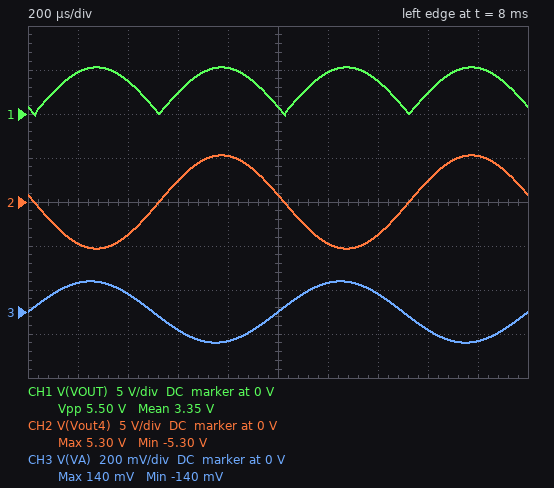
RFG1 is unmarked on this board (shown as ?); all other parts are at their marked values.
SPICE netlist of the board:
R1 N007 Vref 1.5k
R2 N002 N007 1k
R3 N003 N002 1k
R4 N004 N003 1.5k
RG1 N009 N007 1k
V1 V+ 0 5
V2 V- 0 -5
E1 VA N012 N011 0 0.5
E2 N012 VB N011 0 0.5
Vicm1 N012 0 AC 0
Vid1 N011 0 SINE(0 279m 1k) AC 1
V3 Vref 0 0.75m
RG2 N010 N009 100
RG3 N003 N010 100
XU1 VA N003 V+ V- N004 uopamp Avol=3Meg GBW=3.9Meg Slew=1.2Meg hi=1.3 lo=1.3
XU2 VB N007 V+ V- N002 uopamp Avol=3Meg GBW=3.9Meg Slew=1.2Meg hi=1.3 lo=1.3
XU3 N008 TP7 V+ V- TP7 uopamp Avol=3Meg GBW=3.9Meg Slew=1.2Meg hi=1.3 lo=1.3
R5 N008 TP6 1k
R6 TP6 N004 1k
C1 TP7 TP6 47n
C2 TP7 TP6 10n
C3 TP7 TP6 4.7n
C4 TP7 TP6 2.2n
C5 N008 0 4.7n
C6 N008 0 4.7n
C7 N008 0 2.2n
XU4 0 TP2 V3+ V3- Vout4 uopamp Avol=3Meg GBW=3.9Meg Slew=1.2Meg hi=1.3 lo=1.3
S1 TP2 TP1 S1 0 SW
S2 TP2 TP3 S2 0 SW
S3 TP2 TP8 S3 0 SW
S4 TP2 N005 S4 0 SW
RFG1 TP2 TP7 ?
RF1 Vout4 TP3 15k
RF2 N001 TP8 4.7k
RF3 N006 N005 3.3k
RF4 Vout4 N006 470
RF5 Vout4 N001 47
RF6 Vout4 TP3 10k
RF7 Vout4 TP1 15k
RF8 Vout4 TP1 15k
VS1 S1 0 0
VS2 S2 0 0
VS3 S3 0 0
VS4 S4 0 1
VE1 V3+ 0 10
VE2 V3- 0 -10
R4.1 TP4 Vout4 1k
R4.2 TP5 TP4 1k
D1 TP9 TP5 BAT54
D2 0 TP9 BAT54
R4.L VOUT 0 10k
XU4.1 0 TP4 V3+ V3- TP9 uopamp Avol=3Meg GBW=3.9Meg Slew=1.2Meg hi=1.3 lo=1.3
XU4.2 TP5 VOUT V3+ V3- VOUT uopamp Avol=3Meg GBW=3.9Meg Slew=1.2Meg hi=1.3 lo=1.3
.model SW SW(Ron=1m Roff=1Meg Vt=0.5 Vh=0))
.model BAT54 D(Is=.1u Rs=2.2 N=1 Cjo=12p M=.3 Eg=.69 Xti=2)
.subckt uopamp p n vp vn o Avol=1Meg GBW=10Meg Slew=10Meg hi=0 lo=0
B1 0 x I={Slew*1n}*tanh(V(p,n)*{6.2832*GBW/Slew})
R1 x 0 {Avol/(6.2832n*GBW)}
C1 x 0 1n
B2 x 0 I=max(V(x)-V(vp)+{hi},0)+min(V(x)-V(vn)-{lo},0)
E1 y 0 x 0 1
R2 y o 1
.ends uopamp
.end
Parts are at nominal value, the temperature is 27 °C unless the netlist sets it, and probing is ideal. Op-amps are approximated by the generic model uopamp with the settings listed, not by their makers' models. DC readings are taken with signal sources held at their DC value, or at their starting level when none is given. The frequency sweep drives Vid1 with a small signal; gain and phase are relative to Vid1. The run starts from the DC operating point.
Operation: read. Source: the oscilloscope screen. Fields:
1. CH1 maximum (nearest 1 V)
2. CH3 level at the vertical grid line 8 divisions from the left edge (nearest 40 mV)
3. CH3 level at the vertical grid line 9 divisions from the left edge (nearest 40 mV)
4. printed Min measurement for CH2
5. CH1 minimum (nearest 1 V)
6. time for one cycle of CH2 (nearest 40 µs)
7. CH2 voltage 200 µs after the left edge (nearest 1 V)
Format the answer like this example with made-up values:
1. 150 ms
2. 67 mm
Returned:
1. 5 V
2. -80 mV
3. -120 mV
4. -5.30 V
5. 0 V
6. 1.00 ms
7. -5 V
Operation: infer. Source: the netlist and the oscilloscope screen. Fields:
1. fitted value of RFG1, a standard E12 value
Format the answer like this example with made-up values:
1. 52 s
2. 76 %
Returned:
1. 1 kΩ
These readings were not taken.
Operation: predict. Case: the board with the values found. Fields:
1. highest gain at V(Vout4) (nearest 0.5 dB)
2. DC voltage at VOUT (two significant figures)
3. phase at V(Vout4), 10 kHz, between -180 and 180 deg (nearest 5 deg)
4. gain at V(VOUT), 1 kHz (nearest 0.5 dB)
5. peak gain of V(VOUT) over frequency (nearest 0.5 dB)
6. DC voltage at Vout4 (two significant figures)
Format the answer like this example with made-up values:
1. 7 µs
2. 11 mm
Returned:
1. 64.0 dB
2. 2.8 mV
3. 5 deg
4. 62.0 dB
5. 64.0 dB
6. -2.8 mV
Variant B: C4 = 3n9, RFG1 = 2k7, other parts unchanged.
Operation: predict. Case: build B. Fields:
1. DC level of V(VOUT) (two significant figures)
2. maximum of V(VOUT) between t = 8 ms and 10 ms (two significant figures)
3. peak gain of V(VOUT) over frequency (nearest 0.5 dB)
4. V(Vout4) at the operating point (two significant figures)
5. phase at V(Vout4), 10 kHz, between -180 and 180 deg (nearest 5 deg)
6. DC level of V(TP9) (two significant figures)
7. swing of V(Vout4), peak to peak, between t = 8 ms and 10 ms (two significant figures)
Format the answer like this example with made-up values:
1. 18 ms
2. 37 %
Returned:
1. 1.0 mV
2. 2.0 V
3. 55.5 dB
4. -1.0 mV
5. 20 deg
6. 64 mV
7. 3.9 V
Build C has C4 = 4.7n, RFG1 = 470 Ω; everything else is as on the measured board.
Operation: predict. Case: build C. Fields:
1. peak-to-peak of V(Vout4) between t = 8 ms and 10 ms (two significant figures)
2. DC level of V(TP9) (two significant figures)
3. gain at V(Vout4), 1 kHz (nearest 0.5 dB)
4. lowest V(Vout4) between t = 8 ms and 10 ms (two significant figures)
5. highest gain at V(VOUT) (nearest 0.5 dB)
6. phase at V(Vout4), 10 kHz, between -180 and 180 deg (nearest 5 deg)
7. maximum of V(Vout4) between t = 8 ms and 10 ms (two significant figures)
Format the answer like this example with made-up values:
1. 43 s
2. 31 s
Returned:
1. 17 V
2. 110 mV
3. 68.5 dB
4. -8.7 V
5. 69.5 dB
6. -20 deg
7. 8.7 V
